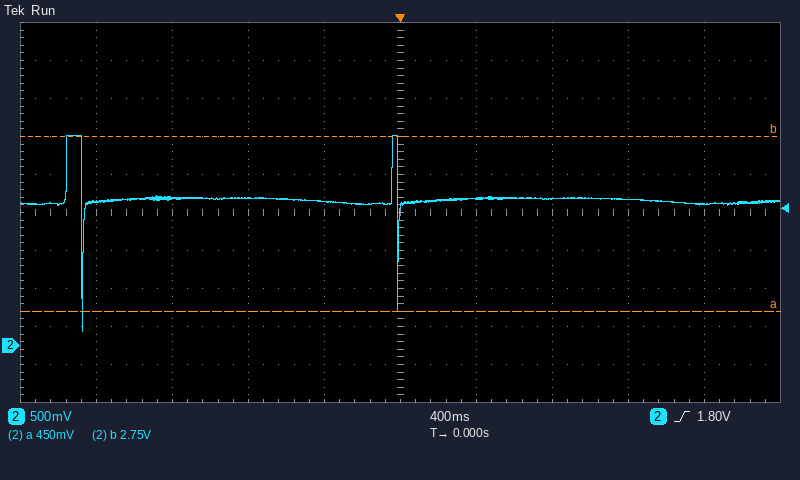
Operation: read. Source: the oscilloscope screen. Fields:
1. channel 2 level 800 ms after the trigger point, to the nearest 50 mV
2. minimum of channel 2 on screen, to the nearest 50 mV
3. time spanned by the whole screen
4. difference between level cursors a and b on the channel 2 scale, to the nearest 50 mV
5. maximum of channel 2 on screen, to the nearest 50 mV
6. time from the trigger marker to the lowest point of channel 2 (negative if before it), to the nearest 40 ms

1.95 V
200 mV
4 s
2.30 V
2.75 V
-1.68 s
